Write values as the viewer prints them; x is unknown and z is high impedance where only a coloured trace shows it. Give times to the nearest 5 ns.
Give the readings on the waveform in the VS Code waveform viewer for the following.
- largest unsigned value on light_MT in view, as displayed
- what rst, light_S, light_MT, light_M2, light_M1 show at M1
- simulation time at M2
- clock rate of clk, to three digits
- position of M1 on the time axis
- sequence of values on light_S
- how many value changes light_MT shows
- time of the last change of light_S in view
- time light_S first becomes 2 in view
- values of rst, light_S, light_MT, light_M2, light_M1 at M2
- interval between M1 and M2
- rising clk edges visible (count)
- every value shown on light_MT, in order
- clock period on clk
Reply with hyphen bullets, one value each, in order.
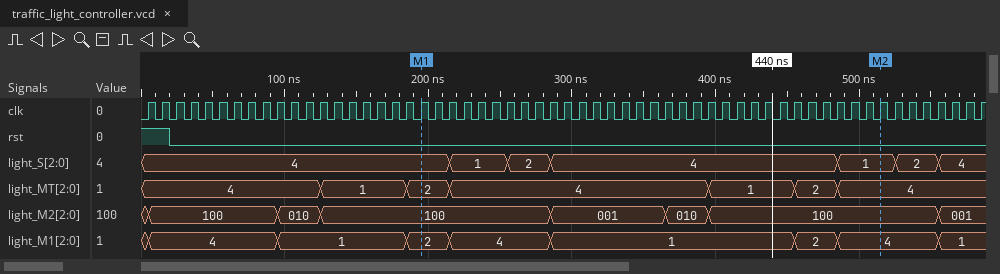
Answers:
- 4
- rst=0, light_S=4, light_MT=2, light_M2=100, light_M1=2
- 515 ns
- 100 MHz
- 195 ns
- 4, 1, 2, 4, 1, 2, 4
- 6
- 555 ns
- 255 ns
- rst=0, light_S=1, light_MT=4, light_M2=100, light_M1=4
- 320 ns
- 59
- 4, 1, 2, 4, 1, 2, 4
- 10 ns
